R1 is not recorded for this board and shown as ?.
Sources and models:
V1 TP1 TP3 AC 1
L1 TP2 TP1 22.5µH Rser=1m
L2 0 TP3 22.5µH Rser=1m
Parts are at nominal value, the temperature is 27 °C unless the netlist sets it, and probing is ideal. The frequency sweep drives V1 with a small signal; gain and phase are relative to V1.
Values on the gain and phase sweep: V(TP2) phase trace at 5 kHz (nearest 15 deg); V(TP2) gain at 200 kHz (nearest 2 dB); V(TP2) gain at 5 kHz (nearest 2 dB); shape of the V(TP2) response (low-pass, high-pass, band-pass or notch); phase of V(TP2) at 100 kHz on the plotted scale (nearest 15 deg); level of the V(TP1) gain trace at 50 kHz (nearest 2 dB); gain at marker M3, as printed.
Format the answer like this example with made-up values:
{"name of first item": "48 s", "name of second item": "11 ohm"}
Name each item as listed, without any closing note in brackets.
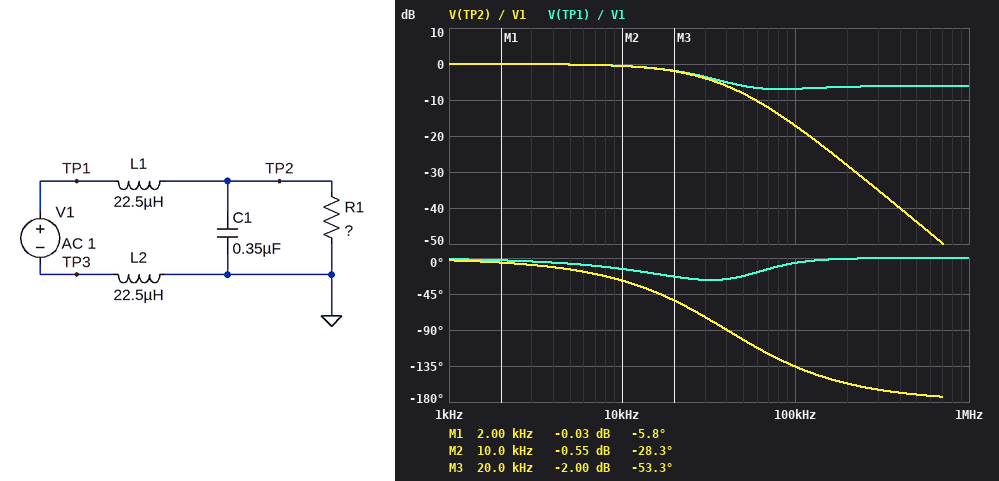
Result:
{"V(TP2) phase trace at 5 kHz": "-15 deg", "V(TP2) gain at 200 kHz": "-28 dB", "V(TP2) gain at 5 kHz": "0 dB", "shape of the V(TP2) response": "low-pass", "phase of V(TP2) at 100 kHz on the plotted scale": "-135 deg", "level of the V(TP1) gain trace at 50 kHz": "-6 dB", "gain at marker M3, as printed": "-2.00 dB"}
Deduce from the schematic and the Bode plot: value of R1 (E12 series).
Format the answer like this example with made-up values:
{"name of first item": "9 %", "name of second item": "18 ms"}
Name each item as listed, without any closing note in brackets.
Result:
{"value of R1": "5.6 Ω"}
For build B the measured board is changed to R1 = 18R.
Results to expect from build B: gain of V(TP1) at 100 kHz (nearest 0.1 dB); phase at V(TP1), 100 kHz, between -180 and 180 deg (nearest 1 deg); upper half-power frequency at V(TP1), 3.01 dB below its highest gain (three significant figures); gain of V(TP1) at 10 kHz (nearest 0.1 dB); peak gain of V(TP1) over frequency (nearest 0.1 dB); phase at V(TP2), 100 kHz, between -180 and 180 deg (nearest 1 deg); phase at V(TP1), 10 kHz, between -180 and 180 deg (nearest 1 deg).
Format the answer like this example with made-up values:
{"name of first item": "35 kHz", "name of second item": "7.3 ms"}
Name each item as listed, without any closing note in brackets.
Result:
{"gain of V(TP1) at 100 kHz": "-7.7 dB", "phase at V(TP1), 100 kHz, between -180 and 180 deg": "-4 deg", "upper half-power frequency at V(TP1), 3.01 dB below its highest gain": "42.1 kHz", "gain of V(TP1) at 10 kHz": "0.2 dB", "peak gain of V(TP1) over frequency": "1.4 dB", "phase at V(TP2), 100 kHz, between -180 and 180 deg": "-163 deg", "phase at V(TP1), 10 kHz, between -180 and 180 deg": "-5 deg"}
